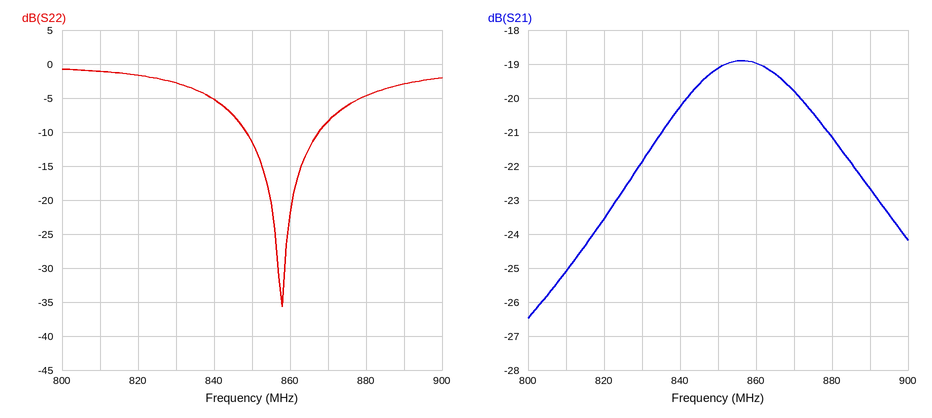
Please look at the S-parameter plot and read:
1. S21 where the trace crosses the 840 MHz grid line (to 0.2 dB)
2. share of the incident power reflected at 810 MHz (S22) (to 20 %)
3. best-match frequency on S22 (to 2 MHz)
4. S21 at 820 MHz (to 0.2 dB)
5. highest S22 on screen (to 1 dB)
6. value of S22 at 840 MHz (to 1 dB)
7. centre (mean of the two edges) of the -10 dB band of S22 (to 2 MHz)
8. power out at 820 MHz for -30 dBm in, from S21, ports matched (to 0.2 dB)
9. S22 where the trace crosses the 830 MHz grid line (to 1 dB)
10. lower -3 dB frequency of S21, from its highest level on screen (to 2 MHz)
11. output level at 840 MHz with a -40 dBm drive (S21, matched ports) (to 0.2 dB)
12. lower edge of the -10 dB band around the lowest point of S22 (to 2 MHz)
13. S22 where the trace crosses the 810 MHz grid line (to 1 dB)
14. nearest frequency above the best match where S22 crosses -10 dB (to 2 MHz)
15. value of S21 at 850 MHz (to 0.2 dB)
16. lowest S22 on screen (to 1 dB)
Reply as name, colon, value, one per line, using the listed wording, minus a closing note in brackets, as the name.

S21 where the trace crosses the 840 MHz grid line: -20.2 dB
share of the incident power reflected at 810 MHz (S22): 80 %
best-match frequency on S22: 858 MHz
S21 at 820 MHz: -23.6 dB
highest S22 on screen: -1 dB
value of S22 at 840 MHz: -5 dB
centre (mean of the two edges) of the -10 dB band of S22: 858 MHz
power out at 820 MHz for -30 dBm in, from S21, ports matched: -53.6 dBm
S22 where the trace crosses the 830 MHz grid line: -3 dB
lower -3 dB frequency of S21, from its highest level on screen: 830 MHz
output level at 840 MHz with a -40 dBm drive (S21, matched ports): -60.2 dBm
lower edge of the -10 dB band around the lowest point of S22: 848 MHz
S22 where the trace crosses the 810 MHz grid line: -1 dB
nearest frequency above the best match where S22 crosses -10 dB: 868 MHz
value of S21 at 850 MHz: -19.2 dB
lowest S22 on screen: -36 dB
